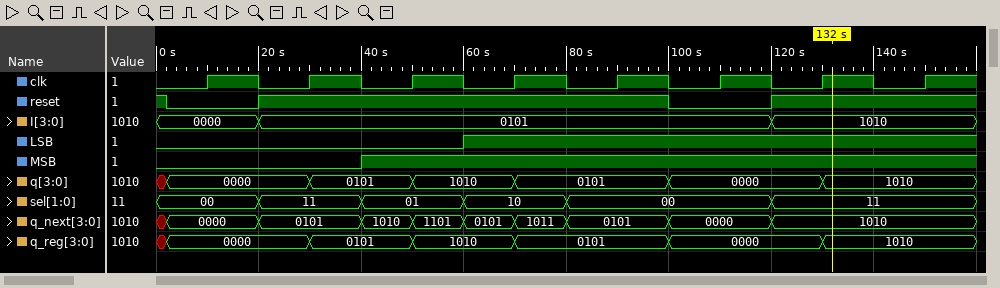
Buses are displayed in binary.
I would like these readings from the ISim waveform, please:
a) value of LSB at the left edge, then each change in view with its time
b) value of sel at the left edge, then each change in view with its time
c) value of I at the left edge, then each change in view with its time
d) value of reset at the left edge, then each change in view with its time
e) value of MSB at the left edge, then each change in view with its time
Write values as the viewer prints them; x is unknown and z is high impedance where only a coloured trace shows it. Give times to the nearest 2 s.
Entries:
0, 1 at 60 s
00, 11 at 20 s, 01 at 40 s, 10 at 60 s, 00 at 80 s, 11 at 120 s
0000, 0101 at 20 s, 1010 at 120 s
1, 0 at 2 s, 1 at 20 s, 0 at 100 s, 1 at 120 s
0, 1 at 40 s
